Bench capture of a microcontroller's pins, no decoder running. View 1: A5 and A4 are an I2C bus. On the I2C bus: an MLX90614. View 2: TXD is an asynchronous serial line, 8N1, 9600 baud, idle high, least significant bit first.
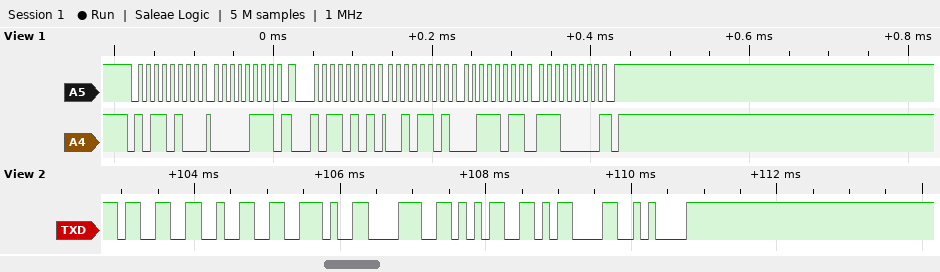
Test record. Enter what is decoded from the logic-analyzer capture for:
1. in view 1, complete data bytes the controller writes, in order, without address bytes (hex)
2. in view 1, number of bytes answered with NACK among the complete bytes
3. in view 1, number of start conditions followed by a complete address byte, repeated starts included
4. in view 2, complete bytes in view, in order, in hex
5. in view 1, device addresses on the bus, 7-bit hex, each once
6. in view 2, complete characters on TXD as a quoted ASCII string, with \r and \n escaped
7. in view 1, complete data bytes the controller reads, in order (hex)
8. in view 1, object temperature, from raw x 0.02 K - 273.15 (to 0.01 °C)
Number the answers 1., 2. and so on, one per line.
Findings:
1. 07
2. 1
3. 2
4. 33 32 2E 38 35 0D 0A
5. 0x5A
6. "32.85\r\n"
7. 2D 3B E0
8. 29.83 °C
